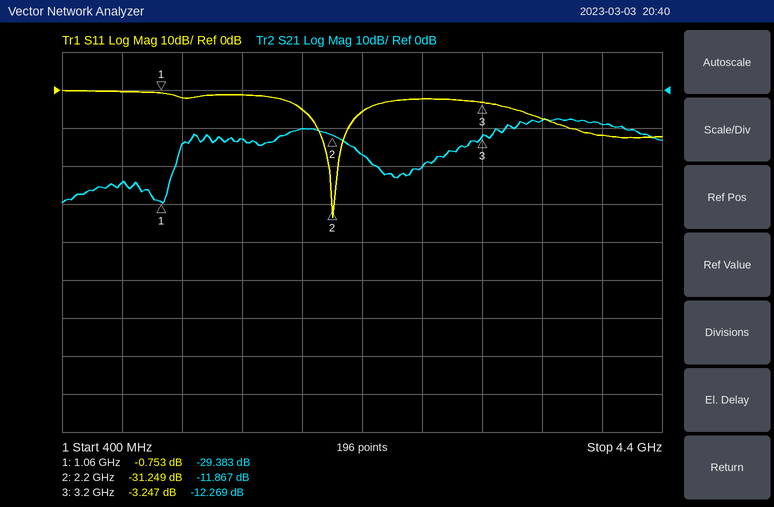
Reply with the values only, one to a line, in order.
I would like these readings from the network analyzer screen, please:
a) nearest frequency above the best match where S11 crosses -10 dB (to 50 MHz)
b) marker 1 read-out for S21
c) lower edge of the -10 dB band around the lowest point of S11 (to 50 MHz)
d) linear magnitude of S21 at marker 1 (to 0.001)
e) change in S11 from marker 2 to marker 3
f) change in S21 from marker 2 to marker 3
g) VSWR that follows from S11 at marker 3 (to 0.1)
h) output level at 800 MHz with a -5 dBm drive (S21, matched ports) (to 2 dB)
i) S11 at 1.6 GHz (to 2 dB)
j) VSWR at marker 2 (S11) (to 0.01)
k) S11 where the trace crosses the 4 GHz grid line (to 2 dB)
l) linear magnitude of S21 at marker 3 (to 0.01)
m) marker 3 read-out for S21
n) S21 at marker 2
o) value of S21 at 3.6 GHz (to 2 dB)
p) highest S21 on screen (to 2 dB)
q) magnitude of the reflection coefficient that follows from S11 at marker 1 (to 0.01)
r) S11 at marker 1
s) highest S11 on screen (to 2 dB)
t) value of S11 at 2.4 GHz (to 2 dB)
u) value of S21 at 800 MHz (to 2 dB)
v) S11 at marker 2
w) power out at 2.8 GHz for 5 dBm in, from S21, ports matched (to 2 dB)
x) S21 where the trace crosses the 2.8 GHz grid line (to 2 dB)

2.30 GHz
-29.383 dB
2.10 GHz
0.034
28.002 dB
-0.402 dB
5.4
-30 dBm
-2 dB
1.06
-12 dB
0.24
-12.269 dB
-11.867 dB
-8 dB
-8 dB
0.92
-0.753 dB
0 dB
-6 dB
-24 dB
-31.249 dB
-16 dBm
-20 dB
